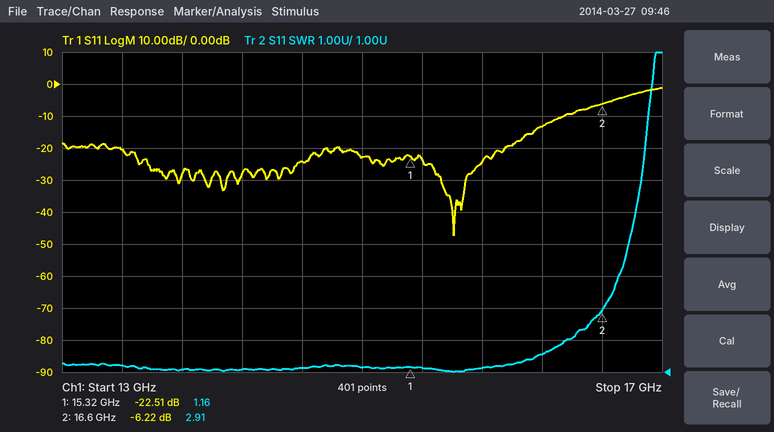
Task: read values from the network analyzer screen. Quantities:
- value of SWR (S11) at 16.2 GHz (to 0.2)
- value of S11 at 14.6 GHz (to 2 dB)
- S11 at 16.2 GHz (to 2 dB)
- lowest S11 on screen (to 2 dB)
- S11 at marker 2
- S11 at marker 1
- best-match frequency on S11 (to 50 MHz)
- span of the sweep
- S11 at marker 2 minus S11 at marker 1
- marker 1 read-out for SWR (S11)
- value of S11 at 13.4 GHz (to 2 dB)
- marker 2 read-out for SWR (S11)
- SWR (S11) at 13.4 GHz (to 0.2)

1.6
-24 dB
-14 dB
-48 dB
-6.22 dB
-22.51 dB
15.60 GHz
4 GHz
16.29 dB
1.16
-20 dB
2.91
1.2
